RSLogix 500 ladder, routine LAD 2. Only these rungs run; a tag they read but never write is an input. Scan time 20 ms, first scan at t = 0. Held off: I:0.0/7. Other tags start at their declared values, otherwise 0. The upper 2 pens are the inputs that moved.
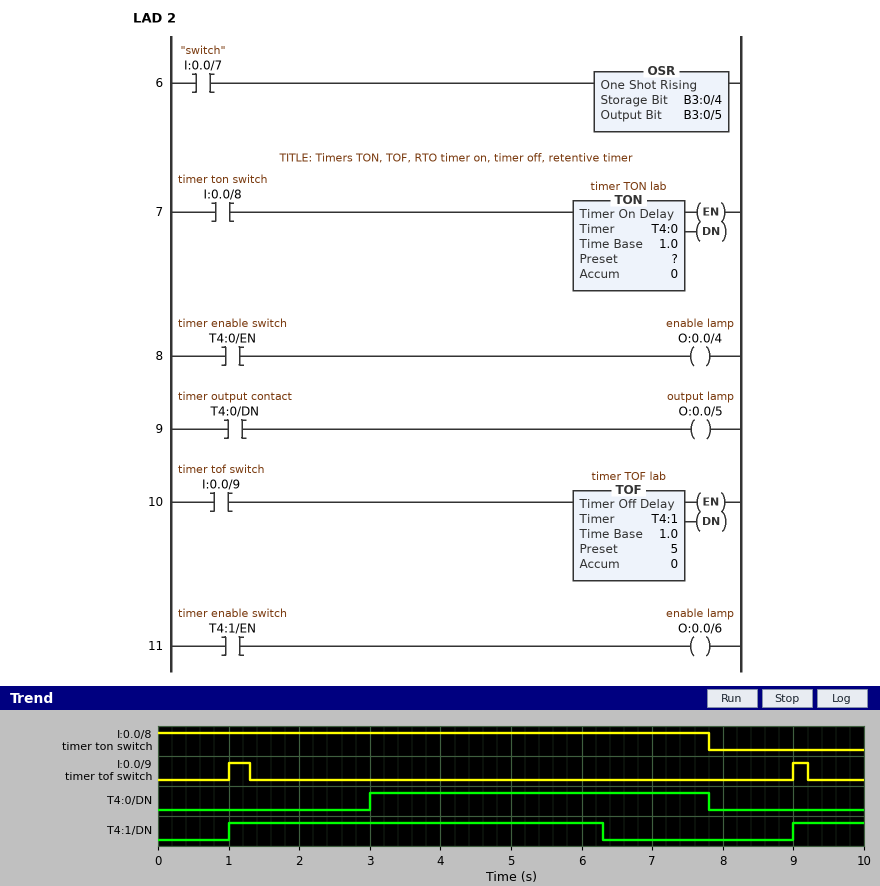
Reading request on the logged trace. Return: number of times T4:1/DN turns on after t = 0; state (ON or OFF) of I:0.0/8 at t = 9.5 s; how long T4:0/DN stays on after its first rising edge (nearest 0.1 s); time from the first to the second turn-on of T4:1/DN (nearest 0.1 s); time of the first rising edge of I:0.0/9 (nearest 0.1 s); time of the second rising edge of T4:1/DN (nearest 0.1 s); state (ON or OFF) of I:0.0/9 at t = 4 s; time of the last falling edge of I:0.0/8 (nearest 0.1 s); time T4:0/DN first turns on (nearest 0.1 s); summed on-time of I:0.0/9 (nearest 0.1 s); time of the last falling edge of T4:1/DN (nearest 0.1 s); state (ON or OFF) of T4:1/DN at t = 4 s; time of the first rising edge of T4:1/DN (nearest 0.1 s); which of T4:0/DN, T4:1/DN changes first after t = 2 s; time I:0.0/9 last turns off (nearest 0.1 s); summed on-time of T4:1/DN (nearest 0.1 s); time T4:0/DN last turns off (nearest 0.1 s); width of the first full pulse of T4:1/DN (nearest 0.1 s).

2
OFF
4.8 s
8.0 s
1.0 s
9.0 s
OFF
7.8 s
3.0 s
0.5 s
6.3 s
ON
1.0 s
T4:0/DN
9.2 s
6.3 s
7.8 s
5.3 s
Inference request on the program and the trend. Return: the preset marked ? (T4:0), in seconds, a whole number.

3 s
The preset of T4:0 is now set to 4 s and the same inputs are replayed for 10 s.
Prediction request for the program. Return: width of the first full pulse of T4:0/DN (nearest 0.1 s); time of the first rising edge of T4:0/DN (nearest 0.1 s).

3.8 s
4.0 s
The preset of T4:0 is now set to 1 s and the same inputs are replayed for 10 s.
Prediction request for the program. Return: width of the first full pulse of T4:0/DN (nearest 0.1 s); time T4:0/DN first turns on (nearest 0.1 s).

6.8 s
1.0 s
